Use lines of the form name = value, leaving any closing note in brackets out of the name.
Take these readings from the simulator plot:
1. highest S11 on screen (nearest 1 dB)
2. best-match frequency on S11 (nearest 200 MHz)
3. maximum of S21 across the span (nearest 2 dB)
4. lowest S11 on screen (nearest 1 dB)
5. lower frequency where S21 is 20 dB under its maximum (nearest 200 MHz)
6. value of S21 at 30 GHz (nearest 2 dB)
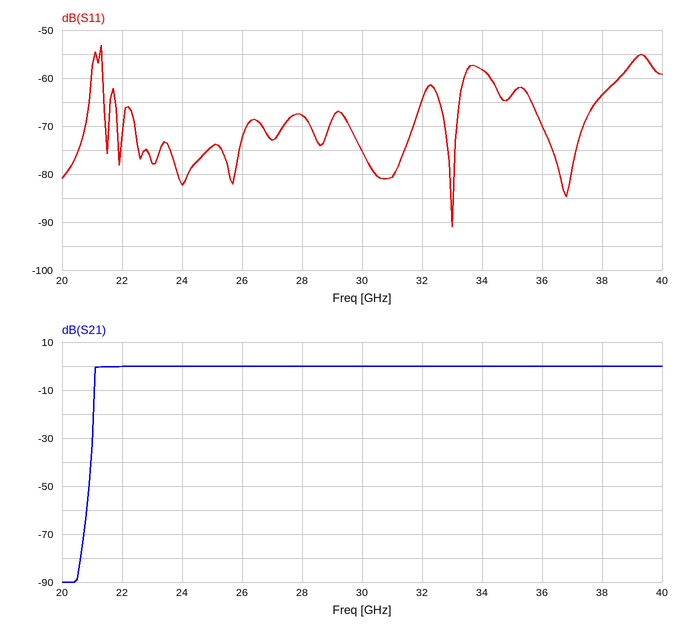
highest S11 on screen = -53 dB
best-match frequency on S11 = 33.0 GHz
maximum of S21 across the span = 0 dB
lowest S11 on screen = -91 dB
lower frequency where S21 is 20 dB under its maximum = 21.0 GHz
value of S21 at 30 GHz = 0 dB
